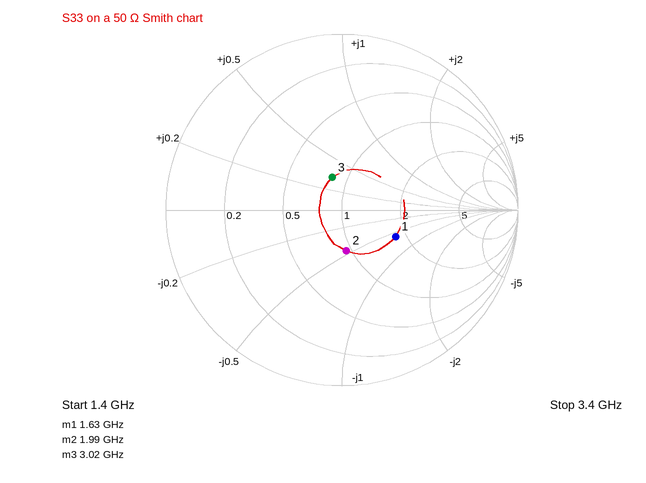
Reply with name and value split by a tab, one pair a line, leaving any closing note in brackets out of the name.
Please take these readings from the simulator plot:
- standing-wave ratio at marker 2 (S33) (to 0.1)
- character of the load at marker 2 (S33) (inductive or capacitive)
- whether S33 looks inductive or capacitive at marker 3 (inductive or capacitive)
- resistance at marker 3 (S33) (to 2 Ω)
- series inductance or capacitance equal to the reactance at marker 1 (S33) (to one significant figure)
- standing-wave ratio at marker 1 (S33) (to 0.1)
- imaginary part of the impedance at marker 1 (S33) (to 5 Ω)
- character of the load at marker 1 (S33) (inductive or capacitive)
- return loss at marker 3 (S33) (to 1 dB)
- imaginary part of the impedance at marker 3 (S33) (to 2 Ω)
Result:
standing-wave ratio at marker 2 (S33)	1.6
character of the load at marker 2 (S33)	capacitive
whether S33 looks inductive or capacitive at marker 3	inductive
resistance at marker 3 (S33)	42 Ω
series inductance or capacitance equal to the reactance at marker 1 (S33)	3 pF
standing-wave ratio at marker 1 (S33)	2.0
imaginary part of the impedance at marker 1 (S33)	-30 Ω
character of the load at marker 1 (S33)	capacitive
return loss at marker 3 (S33)	14 dB
imaginary part of the impedance at marker 3 (S33)	+16 Ω
